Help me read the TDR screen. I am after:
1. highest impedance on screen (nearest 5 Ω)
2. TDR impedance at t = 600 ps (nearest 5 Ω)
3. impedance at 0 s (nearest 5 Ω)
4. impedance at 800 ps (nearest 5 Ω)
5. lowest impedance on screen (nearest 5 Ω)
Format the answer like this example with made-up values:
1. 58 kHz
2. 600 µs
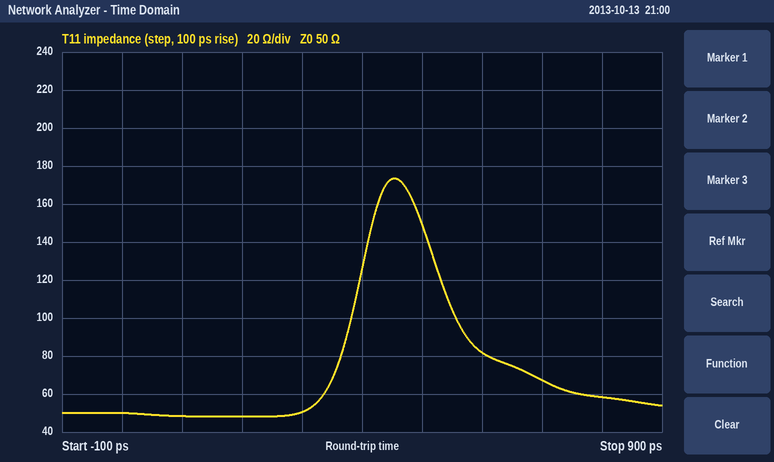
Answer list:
1. 175 Ω
2. 80 Ω
3. 50 Ω
4. 60 Ω
5. 50 Ω
